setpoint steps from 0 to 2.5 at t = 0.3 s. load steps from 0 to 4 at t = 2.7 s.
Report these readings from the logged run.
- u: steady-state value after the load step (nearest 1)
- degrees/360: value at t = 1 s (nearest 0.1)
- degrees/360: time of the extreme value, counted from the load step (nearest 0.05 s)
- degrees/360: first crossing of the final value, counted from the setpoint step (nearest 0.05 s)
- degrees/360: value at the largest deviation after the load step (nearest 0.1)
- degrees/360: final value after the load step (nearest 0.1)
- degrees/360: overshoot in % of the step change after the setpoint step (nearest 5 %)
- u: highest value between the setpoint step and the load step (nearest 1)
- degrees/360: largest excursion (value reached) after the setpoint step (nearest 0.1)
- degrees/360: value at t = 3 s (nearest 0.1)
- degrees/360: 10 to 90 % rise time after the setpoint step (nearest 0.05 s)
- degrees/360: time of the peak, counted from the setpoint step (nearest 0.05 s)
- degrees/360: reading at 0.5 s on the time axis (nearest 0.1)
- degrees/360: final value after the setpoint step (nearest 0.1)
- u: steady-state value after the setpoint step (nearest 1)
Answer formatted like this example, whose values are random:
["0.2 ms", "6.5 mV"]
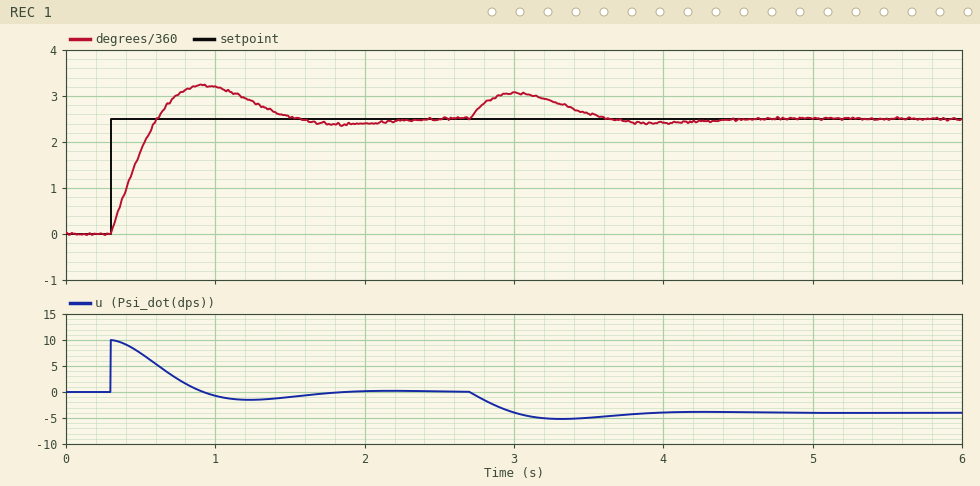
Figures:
["-4", "3.2", "0.30 s", "0.30 s", "3.1", "2.5", "30 %", "10", "3.2", "3.1", "0.25 s", "0.60 s", "1.8", "2.5", "0"]
